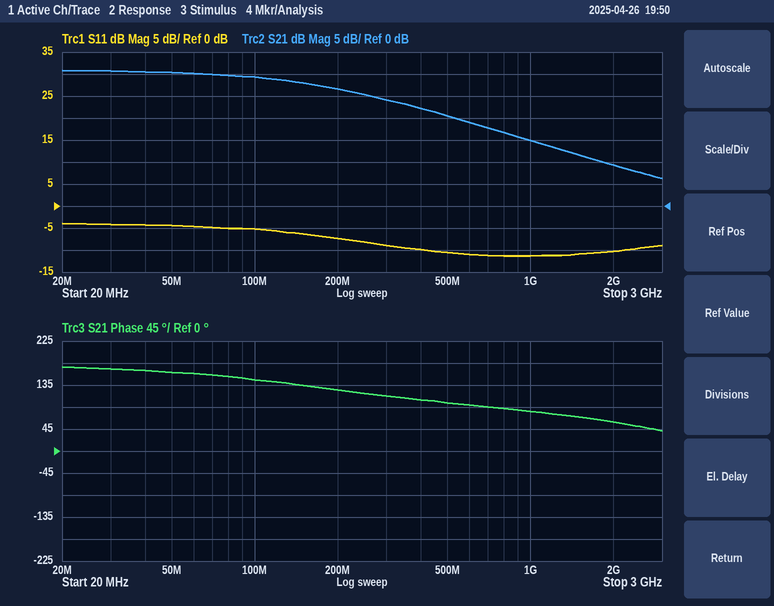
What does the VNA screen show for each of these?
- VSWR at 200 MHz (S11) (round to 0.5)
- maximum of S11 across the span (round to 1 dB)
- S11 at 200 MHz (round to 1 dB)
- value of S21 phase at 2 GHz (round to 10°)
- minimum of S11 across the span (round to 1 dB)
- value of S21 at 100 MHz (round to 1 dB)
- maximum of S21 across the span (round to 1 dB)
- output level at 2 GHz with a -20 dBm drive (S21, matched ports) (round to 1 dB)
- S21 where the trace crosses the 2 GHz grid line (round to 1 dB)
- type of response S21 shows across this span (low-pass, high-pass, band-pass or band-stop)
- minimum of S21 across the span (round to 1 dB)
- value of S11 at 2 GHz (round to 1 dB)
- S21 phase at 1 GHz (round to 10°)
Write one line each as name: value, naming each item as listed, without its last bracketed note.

VSWR at 200 MHz (S11): 2.5
maximum of S11 across the span: -4 dB
S11 at 200 MHz: -7 dB
value of S21 phase at 2 GHz: 60°
minimum of S11 across the span: -11 dB
value of S21 at 100 MHz: 29 dB
maximum of S21 across the span: 31 dB
output level at 2 GHz with a -20 dBm drive (S21, matched ports): -11 dBm
S21 where the trace crosses the 2 GHz grid line: 9 dB
type of response S21 shows across this span: low-pass
minimum of S21 across the span: 6 dB
value of S11 at 2 GHz: -10 dB
S21 phase at 1 GHz: 80°
